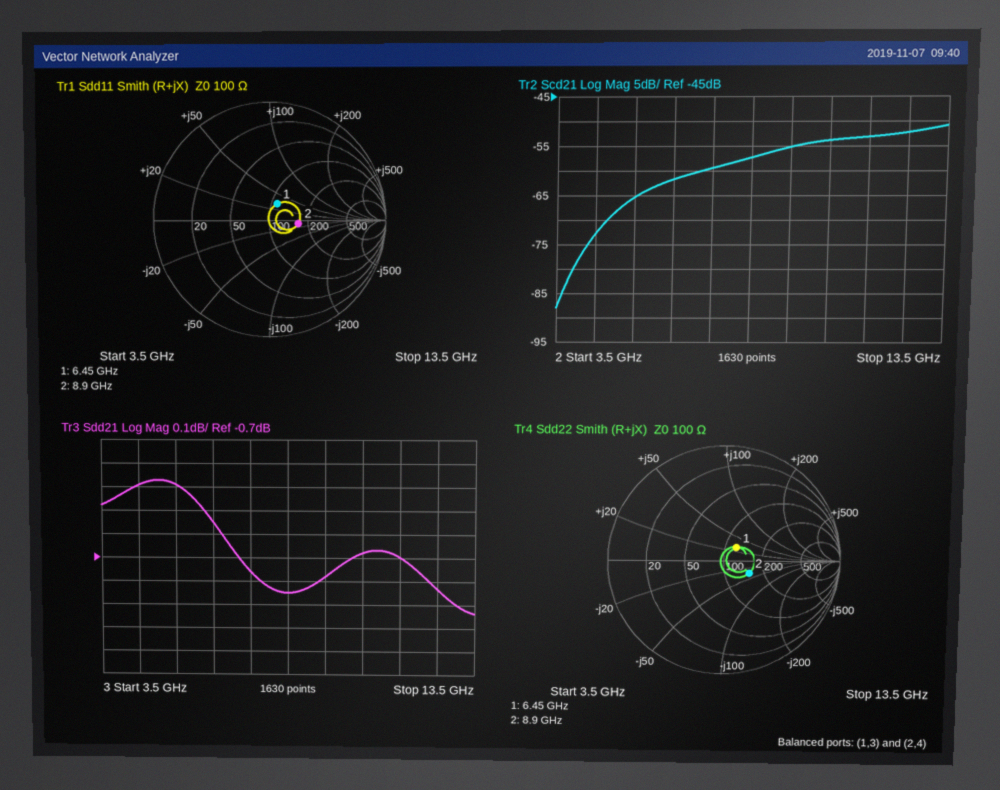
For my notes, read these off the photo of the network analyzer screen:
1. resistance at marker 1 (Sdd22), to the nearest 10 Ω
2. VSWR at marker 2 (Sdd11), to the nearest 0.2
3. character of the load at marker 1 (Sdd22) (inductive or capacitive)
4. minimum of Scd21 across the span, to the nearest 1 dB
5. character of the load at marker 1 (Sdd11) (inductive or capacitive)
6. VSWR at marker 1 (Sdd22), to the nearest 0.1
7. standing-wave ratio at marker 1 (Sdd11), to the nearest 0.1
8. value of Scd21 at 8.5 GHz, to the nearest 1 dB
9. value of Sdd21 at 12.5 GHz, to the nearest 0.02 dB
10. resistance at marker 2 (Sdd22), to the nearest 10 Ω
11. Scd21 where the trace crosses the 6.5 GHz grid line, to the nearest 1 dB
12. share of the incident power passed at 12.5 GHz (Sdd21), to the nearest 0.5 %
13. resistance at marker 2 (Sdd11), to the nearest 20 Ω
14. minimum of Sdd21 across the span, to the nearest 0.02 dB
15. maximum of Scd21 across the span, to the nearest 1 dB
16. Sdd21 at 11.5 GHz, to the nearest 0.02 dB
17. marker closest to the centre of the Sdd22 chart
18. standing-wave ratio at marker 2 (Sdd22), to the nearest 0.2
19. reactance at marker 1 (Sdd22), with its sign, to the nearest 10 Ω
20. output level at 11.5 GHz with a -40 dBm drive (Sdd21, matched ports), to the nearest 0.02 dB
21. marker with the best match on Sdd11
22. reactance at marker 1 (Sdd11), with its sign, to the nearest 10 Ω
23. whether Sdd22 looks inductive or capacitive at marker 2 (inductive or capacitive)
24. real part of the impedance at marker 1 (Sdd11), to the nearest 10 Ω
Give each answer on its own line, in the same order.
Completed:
120 Ω
1.6
inductive
-88 dB
inductive
1.4
1.4
-57 dB
-0.84 dB
150 Ω
-62 dB
82.5 %
160 Ω
-0.94 dB
-51 dB
-0.70 dB
marker 1
1.6
+30 Ω
-40.70 dBm
marker 1
+30 Ω
capacitive
110 Ω
